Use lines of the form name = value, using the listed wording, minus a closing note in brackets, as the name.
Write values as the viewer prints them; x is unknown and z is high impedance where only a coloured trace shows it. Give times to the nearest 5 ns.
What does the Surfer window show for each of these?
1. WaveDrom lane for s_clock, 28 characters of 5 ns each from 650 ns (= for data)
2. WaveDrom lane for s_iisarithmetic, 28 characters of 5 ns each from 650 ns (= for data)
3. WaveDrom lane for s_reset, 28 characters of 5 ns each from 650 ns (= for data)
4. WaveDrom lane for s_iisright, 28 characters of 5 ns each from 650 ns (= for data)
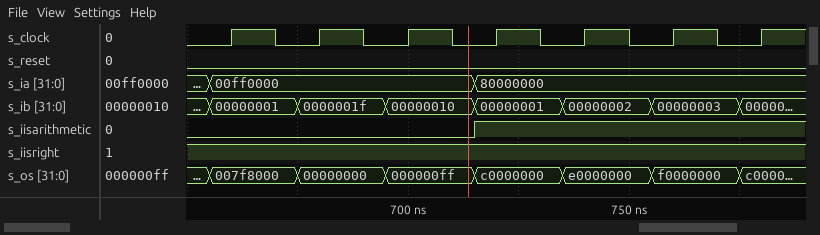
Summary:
WaveDrom lane for s_clock, 28 characters of 5 ns each from 650 ns = {name: 's_clock', wave: '0.1.0.1.0.1.0.1.0.1.0.1.0.1.'}
WaveDrom lane for s_iisarithmetic, 28 characters of 5 ns each from 650 ns = {name: 's_iisarithmetic', wave: '0............1..............'}
WaveDrom lane for s_reset, 28 characters of 5 ns each from 650 ns = {name: 's_reset', wave: '0...........................'}
WaveDrom lane for s_iisright, 28 characters of 5 ns each from 650 ns = {name: 's_iisright', wave: '1...........................'}
